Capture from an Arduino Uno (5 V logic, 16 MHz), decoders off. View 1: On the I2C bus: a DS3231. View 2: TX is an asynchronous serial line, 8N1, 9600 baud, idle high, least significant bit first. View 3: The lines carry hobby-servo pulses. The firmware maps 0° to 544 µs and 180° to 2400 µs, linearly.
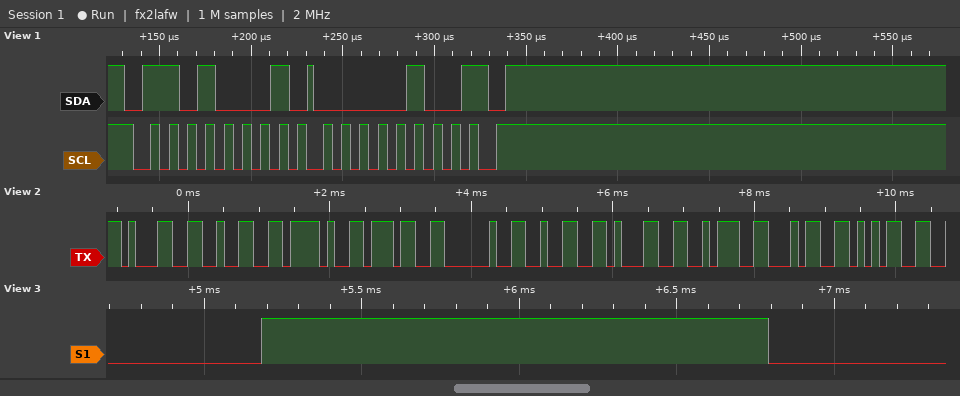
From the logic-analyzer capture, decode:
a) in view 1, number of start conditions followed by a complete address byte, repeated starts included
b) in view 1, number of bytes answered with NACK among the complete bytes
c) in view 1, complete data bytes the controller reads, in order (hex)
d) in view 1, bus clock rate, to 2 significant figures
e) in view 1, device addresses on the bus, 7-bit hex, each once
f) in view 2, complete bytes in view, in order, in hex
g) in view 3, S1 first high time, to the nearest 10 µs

1
1
04
100 kHz
0x68
31 32 2F 37 20 32 31 3A 34 35
1610 µs
